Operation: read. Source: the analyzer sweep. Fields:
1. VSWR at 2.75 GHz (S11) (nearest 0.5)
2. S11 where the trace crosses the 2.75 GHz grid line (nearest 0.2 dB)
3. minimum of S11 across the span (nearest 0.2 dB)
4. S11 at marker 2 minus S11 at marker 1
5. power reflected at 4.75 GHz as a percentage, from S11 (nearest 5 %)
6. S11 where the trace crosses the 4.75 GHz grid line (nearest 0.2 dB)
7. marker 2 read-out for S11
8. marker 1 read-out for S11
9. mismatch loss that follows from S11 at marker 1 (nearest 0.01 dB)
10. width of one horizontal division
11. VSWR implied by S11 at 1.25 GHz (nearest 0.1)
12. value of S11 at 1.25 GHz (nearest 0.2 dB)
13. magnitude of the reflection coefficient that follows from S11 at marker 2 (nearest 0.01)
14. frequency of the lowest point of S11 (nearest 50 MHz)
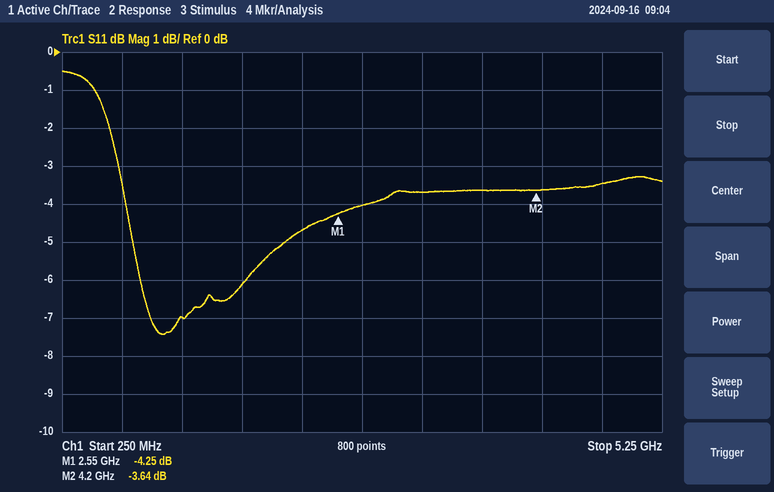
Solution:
4.5
-4.0 dB
-7.4 dB
0.61 dB
45 %
-3.4 dB
-3.64 dB
-4.25 dB
2.05 dB
500 MHz
2.6
-7.0 dB
0.66
1.10 GHz
